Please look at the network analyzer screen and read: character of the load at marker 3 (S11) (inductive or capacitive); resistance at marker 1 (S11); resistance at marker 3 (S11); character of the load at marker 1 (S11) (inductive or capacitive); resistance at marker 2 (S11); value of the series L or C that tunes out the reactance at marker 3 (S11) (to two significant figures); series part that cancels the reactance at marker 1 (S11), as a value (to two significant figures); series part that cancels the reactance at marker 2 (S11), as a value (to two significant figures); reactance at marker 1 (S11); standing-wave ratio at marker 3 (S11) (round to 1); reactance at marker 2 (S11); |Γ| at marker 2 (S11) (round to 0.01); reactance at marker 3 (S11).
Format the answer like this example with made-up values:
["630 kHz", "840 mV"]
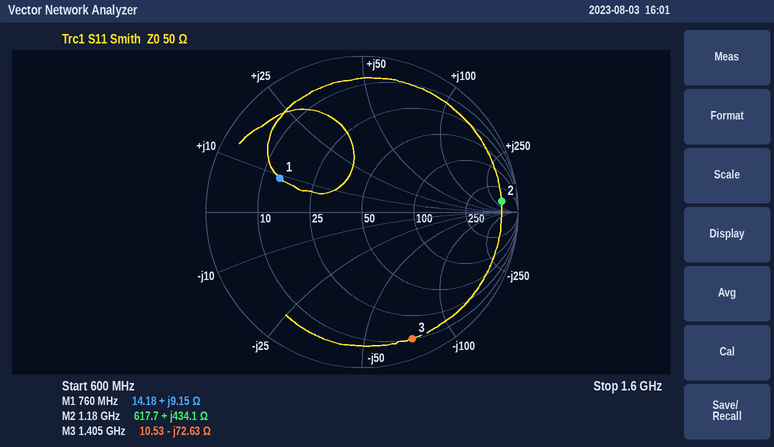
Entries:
["capacitive", "14.18 Ω", "10.53 Ω", "inductive", "617.7 Ω", "8.2 nH", "23 pF", "310 fF", "+9.15 Ω", "15", "+434.1 Ω", "0.90", "-72.63 Ω"]
